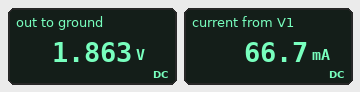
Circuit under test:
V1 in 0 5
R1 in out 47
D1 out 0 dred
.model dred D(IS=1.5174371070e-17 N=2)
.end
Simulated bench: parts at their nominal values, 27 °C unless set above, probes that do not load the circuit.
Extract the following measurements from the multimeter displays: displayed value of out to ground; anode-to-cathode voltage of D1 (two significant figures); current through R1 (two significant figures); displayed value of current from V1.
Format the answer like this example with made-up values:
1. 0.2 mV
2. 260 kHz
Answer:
1. 1.863 V
2. 1.9 V
3. 67 mA
4. 66.7 mA
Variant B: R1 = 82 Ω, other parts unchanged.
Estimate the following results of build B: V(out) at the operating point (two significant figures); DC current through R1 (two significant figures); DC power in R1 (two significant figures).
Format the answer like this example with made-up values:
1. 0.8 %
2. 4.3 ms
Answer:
1. 1.8 V
2. 39 mA
3. 120 mW
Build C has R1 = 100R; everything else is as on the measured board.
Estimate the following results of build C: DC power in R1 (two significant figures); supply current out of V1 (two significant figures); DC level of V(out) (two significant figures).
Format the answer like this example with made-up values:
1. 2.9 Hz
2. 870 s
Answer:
1. 100 mW
2. 32 mA
3. 1.8 V
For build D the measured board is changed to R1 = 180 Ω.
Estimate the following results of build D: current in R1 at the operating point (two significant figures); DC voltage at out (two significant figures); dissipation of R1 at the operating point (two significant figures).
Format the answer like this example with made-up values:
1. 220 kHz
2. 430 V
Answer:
1. 18 mA
2. 1.8 V
3. 57 mW
